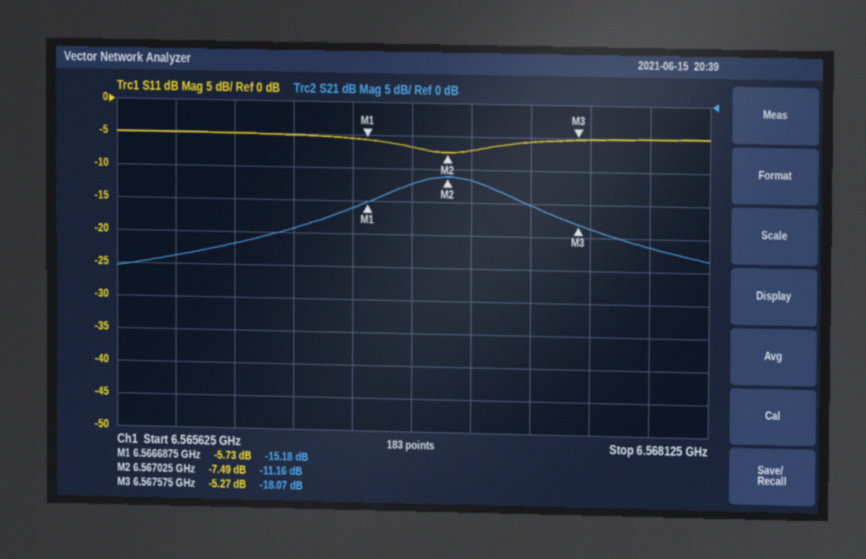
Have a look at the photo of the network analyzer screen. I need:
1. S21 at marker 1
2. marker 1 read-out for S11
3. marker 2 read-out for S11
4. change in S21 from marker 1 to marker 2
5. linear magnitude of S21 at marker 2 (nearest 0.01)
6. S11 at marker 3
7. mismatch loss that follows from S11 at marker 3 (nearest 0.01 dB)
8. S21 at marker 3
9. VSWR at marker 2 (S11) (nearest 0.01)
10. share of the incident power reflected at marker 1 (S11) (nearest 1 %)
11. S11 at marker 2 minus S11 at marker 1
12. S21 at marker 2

-15.18 dB
-5.73 dB
-7.49 dB
4.02 dB
0.28
-5.27 dB
1.53 dB
-18.07 dB
2.46
27 %
-1.76 dB
-11.16 dB
